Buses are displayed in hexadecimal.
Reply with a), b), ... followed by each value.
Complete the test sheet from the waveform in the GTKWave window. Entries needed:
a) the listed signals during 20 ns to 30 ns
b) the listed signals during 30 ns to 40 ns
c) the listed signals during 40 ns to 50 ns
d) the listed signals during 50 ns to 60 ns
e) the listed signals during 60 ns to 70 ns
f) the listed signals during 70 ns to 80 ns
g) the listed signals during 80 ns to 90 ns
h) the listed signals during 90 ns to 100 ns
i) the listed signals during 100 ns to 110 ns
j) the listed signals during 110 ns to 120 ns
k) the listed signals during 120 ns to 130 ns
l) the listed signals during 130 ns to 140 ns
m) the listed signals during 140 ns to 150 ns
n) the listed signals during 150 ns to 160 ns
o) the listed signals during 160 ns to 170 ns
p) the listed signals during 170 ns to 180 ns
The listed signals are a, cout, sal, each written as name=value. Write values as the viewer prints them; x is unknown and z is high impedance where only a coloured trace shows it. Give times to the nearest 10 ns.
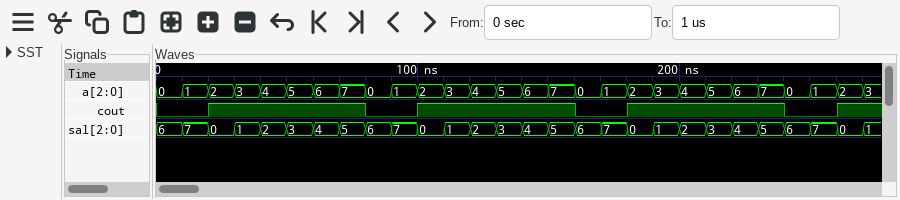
a) a=2, cout=1, sal=0
b) a=3, cout=1, sal=1
c) a=4, cout=1, sal=2
d) a=5, cout=1, sal=3
e) a=6, cout=1, sal=4
f) a=7, cout=1, sal=5
g) a=0, cout=0, sal=6
h) a=1, cout=0, sal=7
i) a=2, cout=1, sal=0
j) a=3, cout=1, sal=1
k) a=4, cout=1, sal=2
l) a=5, cout=1, sal=3
m) a=6, cout=1, sal=4
n) a=7, cout=1, sal=5
o) a=0, cout=0, sal=6
p) a=1, cout=0, sal=7
